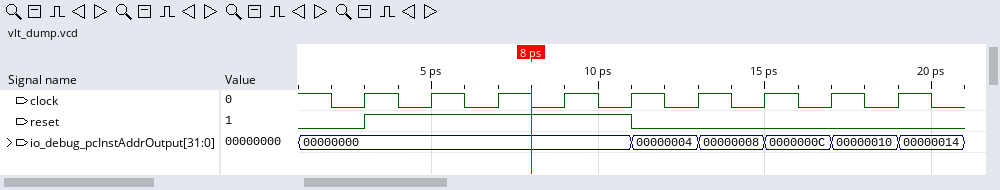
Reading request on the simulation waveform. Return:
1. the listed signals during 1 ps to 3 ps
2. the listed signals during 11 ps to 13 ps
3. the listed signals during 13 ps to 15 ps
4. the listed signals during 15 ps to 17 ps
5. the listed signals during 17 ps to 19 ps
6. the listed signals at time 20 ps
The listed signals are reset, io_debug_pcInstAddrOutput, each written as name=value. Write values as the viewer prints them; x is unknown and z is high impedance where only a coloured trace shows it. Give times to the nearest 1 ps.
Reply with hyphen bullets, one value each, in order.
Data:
- reset=0, io_debug_pcInstAddrOutput=00000000
- reset=0, io_debug_pcInstAddrOutput=00000004
- reset=0, io_debug_pcInstAddrOutput=00000008
- reset=0, io_debug_pcInstAddrOutput=0000000C
- reset=0, io_debug_pcInstAddrOutput=00000010
- reset=0, io_debug_pcInstAddrOutput=00000014
